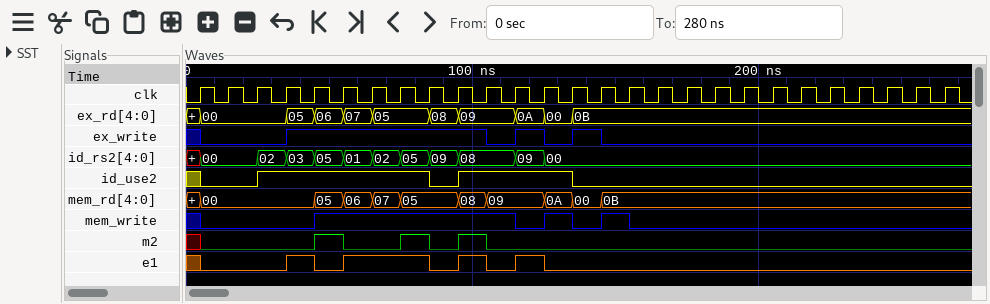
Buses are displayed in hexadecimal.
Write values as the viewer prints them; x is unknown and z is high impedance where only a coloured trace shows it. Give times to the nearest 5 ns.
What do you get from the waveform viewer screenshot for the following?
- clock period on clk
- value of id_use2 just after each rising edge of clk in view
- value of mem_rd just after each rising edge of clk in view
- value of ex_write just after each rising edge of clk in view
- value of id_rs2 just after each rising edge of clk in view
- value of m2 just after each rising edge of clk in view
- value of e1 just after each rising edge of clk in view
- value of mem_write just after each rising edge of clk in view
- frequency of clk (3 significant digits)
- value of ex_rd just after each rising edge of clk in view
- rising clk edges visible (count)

10 ns
0 0 1 1 1 1 1 1 0 1 1 1 1 0 0 0 0 0 0 0 0 0 0 0 0 0 0
00, 00, 00, 00, 05, 06, 07, 05, 05, 08, 09, 09, 0A, 00, 0B, 0B, 0B, 0B, 0B, 0B, 0B, 0B, 0B, 0B, 0B, 0B, 0B
0 0 0 1 1 1 1 1 1 1 0 1 0 1 0 0 0 0 0 0 0 0 0 0 0 0 0
00, 00, 02, 03, 05, 01, 02, 05, 09, 08, 08, 09, 00, 00, 00, 00, 00, 00, 00, 00, 00, 00, 00, 00, 00, 00, 00
0 0 0 0 1 0 0 1 0 1 0 0 0 0 0 0 0 0 0 0 0 0 0 0 0 0 0
0 0 0 1 0 1 1 1 0 1 0 1 0 0 0 0 0 0 0 0 0 0 0 0 0 0 0
0 0 0 0 1 1 1 1 1 1 1 0 1 0 1 0 0 0 0 0 0 0 0 0 0 0 0
100 MHz
00, 00, 00, 05, 06, 07, 05, 05, 08, 09, 09, 0A, 00, 0B, 0B, 0B, 0B, 0B, 0B, 0B, 0B, 0B, 0B, 0B, 0B, 0B, 0B
27
